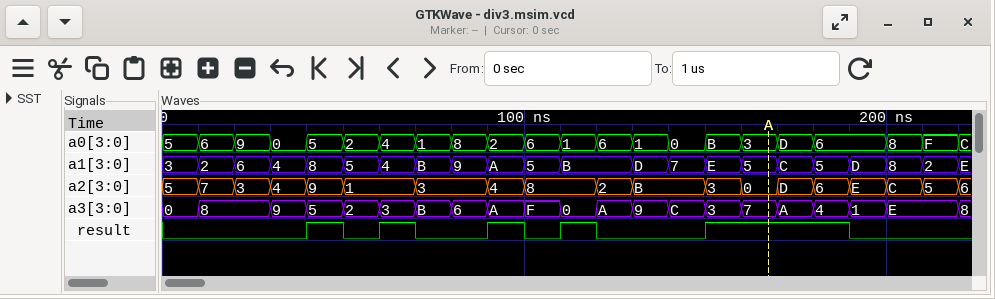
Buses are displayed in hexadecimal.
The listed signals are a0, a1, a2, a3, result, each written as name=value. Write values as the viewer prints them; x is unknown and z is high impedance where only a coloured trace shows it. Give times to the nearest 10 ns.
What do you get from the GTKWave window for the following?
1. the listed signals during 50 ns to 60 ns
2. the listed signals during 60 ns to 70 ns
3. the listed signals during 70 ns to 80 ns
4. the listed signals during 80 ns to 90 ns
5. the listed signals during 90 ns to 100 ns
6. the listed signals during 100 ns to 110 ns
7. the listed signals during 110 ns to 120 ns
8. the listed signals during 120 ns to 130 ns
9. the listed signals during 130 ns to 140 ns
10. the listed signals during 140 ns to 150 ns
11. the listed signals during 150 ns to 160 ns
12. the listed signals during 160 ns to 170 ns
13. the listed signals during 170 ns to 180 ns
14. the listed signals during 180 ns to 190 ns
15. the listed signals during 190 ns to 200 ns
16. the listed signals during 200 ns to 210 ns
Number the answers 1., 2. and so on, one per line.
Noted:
1. a0=2, a1=5, a2=1, a3=2, result=0
2. a0=4, a1=4, a2=1, a3=3, result=1
3. a0=1, a1=B, a2=3, a3=B, result=0
4. a0=8, a1=9, a2=3, a3=6, result=0
5. a0=2, a1=A, a2=4, a3=A, result=1
6. a0=6, a1=5, a2=8, a3=F, result=0
7. a0=1, a1=B, a2=8, a3=0, result=1
8. a0=6, a1=B, a2=2, a3=A, result=0
9. a0=1, a1=D, a2=B, a3=9, result=0
10. a0=0, a1=7, a2=B, a3=C, result=0
11. a0=B, a1=E, a2=3, a3=3, result=1
12. a0=3, a1=5, a2=0, a3=7, result=1
13. a0=D, a1=C, a2=D, a3=A, result=1
14. a0=6, a1=5, a2=6, a3=4, result=1
15. a0=6, a1=D, a2=E, a3=1, result=0
16. a0=8, a1=8, a2=C, a3=E, result=0
